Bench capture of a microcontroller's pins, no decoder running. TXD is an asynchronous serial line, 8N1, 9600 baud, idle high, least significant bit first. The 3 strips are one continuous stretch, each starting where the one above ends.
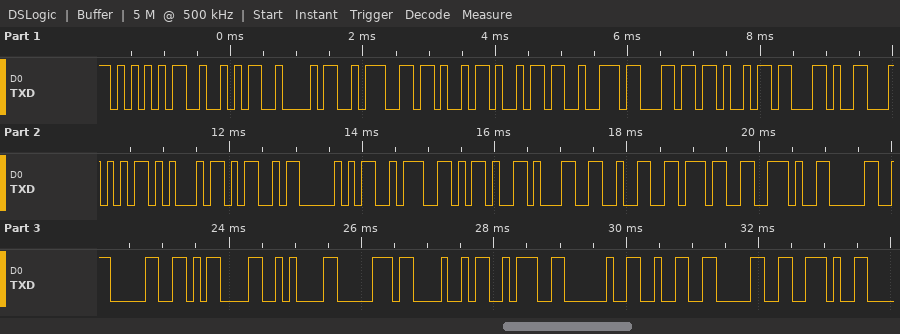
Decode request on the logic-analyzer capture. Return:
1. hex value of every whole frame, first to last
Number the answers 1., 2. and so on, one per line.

1. 0x55 0x52 0x42 0x3A 0x4B 0x69 0x72 0x6C 0x69 0x2C 0x54 0x45 0x4D 0x50 0x3A 0x2D 0x31 0x32 0x37 0x2E 0x30 0x30 0x0D 0x0A 0x70 0x48 0x3A 0x20 0x32 0x30 0x2E
